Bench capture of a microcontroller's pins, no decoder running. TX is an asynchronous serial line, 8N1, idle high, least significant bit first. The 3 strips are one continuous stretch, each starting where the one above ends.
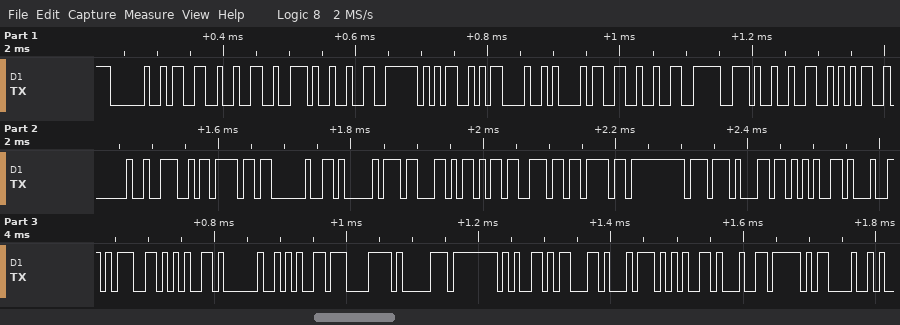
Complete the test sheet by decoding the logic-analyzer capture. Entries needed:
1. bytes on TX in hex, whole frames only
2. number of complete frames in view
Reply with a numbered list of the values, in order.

1. 0x20 0x33 0x32 0x2E 0x32 0x35 0x0D 0x0A 0x33 0x32 0x2E 0x32 0x35 0x20 0x4E 0x6F 0x20 0x41 0x63 0x6B 0x6E 0x6F 0x77 0x6C 0x65 0x64 0x67 0x65 0x20 0x65 0x78 0x70 0x65 0x63 0x74 0x65 0x64 0x0D
2. 38
